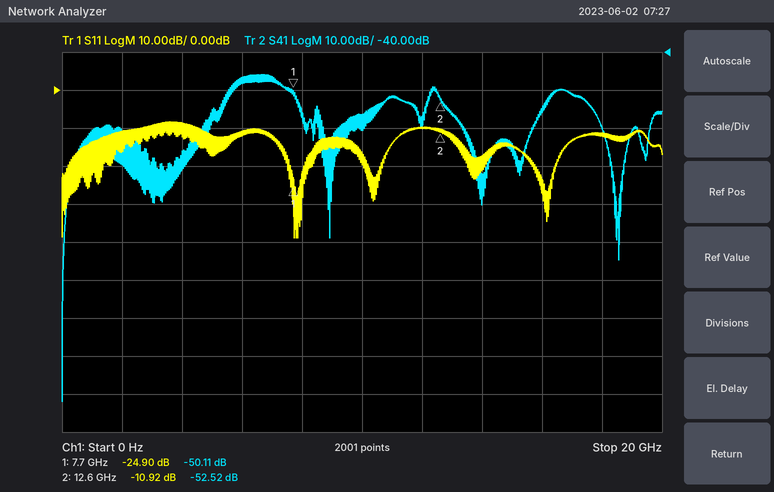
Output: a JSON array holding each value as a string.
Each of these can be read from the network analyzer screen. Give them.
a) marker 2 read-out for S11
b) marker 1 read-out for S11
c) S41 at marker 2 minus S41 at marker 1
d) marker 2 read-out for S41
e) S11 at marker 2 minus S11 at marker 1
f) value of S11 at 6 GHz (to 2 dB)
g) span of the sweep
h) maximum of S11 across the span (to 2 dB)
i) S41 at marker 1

["-10.92 dB", "-24.90 dB", "-2.41 dB", "-52.52 dB", "13.98 dB", "-12 dB", "20 GHz", "-8 dB", "-50.11 dB"]
